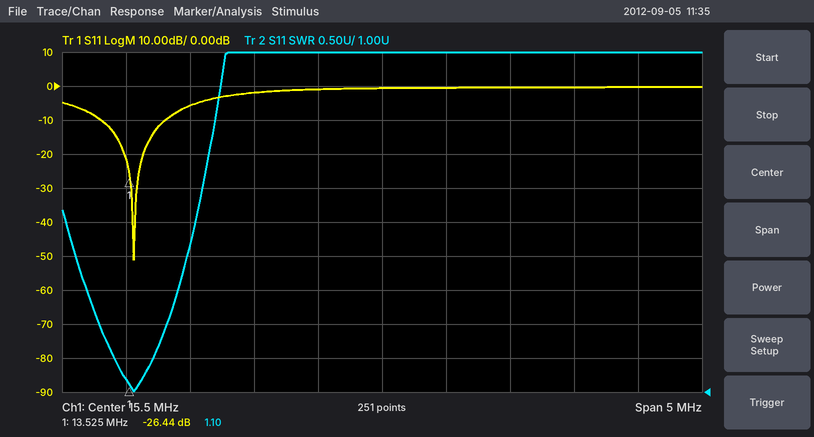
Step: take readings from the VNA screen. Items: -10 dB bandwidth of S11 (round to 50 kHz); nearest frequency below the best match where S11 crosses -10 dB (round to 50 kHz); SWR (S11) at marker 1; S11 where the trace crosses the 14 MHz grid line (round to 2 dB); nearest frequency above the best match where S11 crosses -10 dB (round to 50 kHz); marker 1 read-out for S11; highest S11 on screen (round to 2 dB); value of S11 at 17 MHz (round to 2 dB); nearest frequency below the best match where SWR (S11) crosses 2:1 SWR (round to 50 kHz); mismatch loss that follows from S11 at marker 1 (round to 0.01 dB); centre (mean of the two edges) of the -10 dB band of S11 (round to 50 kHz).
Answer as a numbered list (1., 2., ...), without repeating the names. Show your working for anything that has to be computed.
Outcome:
1. 13.80 MHz − 13.30 MHz = 500 kHz
2. 13.30 MHz
3. 1.10
4. -6 dB
5. 13.80 MHz
6. -26.44 dB
7. 0 dB
8. 0 dB
9. 13.30 MHz
10. −10 log10(1 − 10^(-26.44/10)) ≈ 0.01 dB
11. 13.55 MHz
